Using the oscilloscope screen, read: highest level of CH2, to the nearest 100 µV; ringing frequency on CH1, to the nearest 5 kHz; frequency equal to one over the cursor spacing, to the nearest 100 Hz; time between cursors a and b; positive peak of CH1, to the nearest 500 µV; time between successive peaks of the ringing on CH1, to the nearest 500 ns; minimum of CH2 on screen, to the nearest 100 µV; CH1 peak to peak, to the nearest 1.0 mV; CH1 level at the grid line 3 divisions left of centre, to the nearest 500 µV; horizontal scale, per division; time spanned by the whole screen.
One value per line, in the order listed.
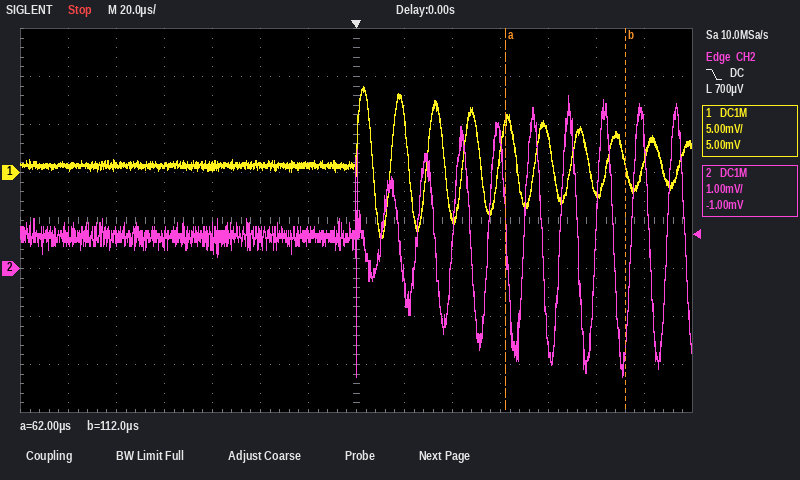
3.6 mV
65 kHz
20.0 kHz
50 µs
9.0 mV
15.0 µs
-2.2 mV
16.0 mV
500 µV
20 µs
280 µs
